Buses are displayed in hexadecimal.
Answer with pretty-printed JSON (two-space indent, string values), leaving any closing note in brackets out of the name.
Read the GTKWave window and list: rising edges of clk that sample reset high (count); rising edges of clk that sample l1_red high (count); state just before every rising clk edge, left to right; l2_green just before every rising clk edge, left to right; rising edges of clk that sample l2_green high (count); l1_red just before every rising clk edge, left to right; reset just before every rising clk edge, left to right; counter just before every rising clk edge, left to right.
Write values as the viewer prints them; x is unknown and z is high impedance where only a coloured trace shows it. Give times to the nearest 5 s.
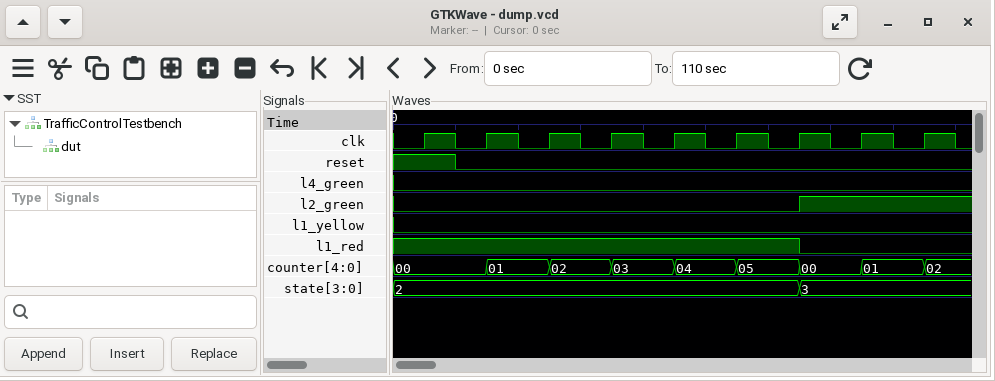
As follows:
{
  "rising edges of clk that sample reset high": "1",
  "rising edges of clk that sample l1_red high": "7",
  "state just before every rising clk edge, left to right": "2, 2, 2, 2, 2, 2, 2, 3, 3",
  "l2_green just before every rising clk edge, left to right": "0 0 0 0 0 0 0 1 1",
  "rising edges of clk that sample l2_green high": "2",
  "l1_red just before every rising clk edge, left to right": "1 1 1 1 1 1 1 0 0",
  "reset just before every rising clk edge, left to right": "1 0 0 0 0 0 0 0 0",
  "counter just before every rising clk edge, left to right": "00, 00, 01, 02, 03, 04, 05, 00, 01"
}
